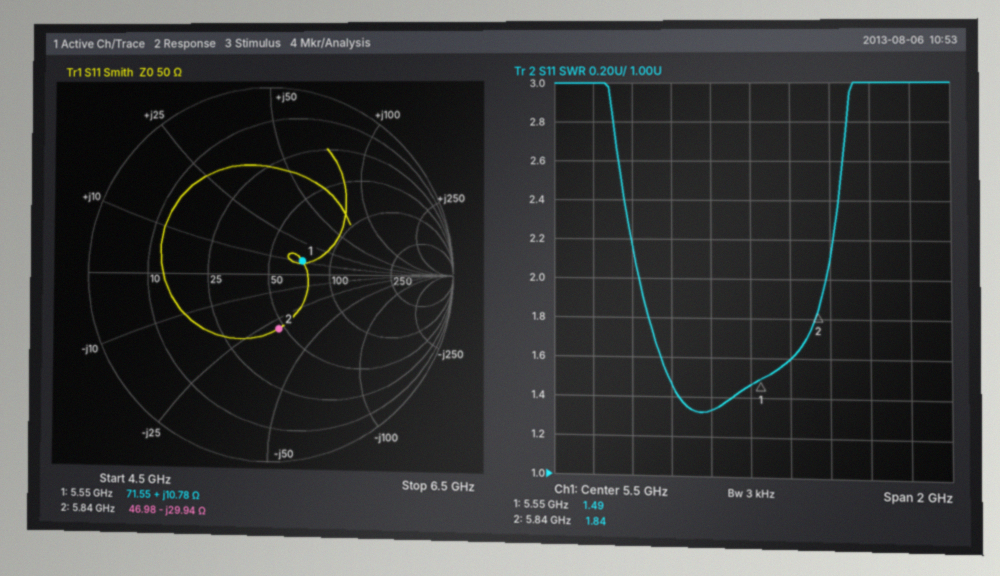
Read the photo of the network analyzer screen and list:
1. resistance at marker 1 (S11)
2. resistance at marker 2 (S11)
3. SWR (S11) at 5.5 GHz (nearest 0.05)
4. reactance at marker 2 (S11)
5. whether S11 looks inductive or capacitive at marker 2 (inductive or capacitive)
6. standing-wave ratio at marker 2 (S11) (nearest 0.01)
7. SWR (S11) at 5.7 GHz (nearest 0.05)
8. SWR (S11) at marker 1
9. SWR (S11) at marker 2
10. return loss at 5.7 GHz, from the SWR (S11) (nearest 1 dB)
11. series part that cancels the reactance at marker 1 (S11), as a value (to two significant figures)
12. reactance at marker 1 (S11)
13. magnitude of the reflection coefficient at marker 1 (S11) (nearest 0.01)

71.55 Ω
46.98 Ω
1.45
-29.94 Ω
capacitive
1.84
1.60
1.49
1.84
13 dB
2.7 pF
+10.78 Ω
0.20
